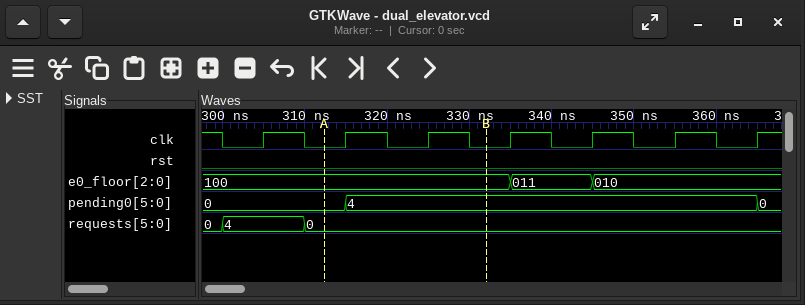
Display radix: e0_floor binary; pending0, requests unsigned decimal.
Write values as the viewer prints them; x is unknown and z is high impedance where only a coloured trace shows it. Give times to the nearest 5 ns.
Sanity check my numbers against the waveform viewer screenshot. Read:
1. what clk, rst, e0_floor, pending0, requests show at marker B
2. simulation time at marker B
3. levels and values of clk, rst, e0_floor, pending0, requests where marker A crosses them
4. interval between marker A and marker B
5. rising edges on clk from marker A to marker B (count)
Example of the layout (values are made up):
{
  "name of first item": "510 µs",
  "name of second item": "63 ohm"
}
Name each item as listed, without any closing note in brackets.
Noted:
{
  "what clk, rst, e0_floor, pending0, requests show at marker B": "clk=0, rst=0, e0_floor=100, pending0=4, requests=0",
  "simulation time at marker B": "330 ns",
  "levels and values of clk, rst, e0_floor, pending0, requests where marker A crosses them": "clk=0, rst=0, e0_floor=100, pending0=0, requests=0",
  "interval between marker A and marker B": "20 ns",
  "rising edges on clk from marker A to marker B": "2"
}
